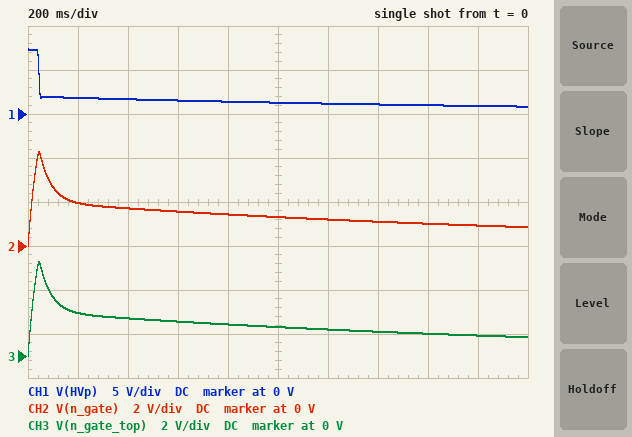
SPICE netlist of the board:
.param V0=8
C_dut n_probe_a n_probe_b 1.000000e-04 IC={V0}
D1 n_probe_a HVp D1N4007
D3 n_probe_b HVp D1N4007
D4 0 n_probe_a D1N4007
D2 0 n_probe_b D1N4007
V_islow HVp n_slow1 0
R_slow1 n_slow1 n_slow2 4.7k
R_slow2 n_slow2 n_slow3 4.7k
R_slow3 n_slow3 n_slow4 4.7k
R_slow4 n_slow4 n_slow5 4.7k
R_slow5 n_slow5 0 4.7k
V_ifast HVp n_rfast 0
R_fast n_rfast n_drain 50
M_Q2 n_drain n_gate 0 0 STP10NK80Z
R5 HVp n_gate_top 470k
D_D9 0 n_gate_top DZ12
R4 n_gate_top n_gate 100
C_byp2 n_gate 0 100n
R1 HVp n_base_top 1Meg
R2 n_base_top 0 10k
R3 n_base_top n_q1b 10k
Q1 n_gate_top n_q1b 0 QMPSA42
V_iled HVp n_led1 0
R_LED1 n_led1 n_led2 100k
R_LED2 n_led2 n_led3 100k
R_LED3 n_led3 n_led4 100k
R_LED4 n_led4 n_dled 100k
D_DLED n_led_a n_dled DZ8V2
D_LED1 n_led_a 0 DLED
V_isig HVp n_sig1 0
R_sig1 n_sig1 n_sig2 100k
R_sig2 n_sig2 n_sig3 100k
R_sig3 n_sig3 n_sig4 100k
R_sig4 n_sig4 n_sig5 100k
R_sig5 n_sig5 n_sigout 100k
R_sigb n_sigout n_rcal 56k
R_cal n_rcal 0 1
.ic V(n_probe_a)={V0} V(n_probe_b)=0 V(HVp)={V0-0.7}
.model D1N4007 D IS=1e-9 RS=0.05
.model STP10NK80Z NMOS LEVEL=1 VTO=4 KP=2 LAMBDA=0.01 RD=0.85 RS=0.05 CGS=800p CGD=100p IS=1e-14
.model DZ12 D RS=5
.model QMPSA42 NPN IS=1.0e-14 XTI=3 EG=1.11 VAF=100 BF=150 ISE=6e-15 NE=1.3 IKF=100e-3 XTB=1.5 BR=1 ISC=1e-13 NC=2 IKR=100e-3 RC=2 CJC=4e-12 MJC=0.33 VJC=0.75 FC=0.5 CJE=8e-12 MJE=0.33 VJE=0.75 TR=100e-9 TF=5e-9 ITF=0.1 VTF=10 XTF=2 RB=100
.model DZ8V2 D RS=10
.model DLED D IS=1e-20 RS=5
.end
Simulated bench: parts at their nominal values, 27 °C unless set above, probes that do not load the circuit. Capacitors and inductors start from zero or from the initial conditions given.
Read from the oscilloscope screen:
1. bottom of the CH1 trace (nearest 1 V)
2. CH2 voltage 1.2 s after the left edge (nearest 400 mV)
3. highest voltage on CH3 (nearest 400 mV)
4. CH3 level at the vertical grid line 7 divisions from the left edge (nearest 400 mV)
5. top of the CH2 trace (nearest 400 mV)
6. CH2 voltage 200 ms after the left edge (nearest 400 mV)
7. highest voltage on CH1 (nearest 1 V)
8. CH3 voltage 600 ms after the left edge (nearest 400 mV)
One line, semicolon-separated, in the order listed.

1 V; 1.2 V; 4.4 V; 1.2 V; 4.4 V; 2.0 V; 7 V; 1.6 V
